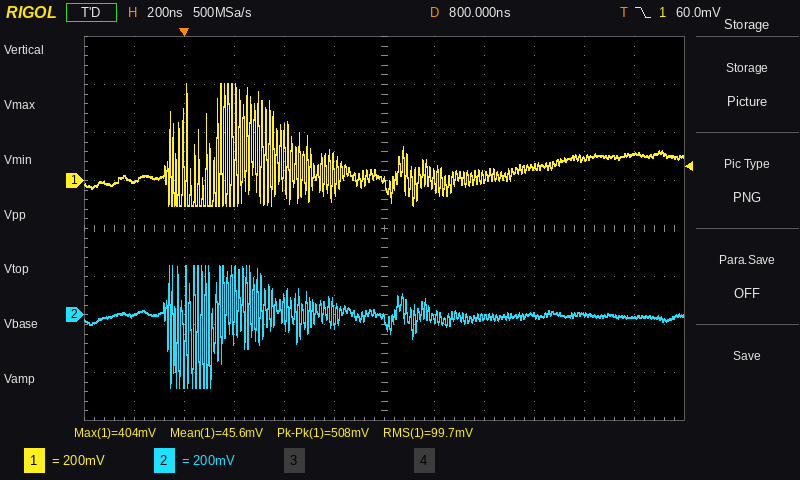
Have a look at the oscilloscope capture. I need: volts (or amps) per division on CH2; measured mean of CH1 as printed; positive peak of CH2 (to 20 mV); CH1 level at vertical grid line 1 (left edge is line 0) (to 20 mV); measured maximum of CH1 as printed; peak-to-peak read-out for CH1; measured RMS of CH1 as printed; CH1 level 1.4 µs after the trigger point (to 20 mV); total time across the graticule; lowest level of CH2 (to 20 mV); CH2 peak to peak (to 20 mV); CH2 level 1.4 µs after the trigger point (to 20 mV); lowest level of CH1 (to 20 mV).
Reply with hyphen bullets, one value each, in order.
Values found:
- 200 mV
- 45.6 mV
- 200 mV
- 0 mV
- 404 mV
- 508 mV
- 99.7 mV
- 60 mV
- 2.4 µs
- -300 mV
- 500 mV
- 0 mV
- -100 mV
